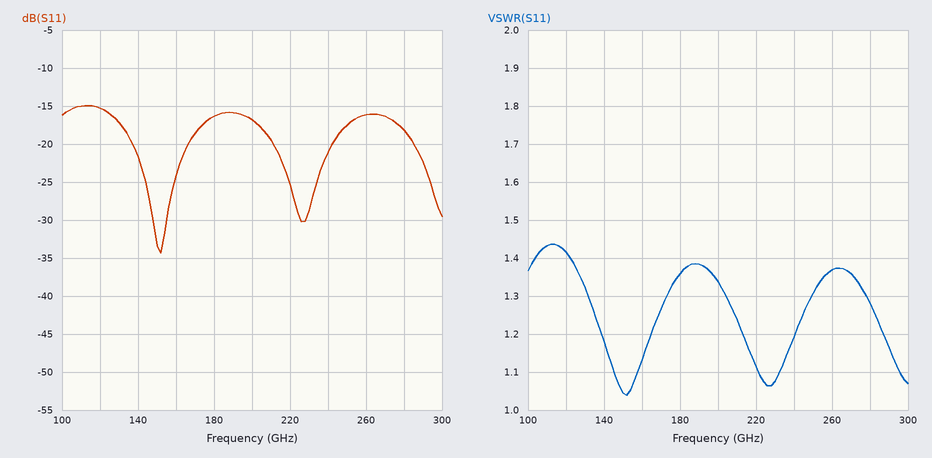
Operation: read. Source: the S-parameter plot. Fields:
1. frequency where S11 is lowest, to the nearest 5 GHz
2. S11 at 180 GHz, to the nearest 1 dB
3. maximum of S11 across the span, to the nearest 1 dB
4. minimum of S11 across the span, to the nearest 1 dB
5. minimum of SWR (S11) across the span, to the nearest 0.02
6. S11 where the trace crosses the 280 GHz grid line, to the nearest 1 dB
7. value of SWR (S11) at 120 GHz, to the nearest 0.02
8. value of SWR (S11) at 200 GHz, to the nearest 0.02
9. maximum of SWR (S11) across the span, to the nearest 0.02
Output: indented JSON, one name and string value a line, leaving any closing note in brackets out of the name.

{
  "frequency where S11 is lowest, to the nearest 5 GHz": "150 GHz",
  "S11 at 180 GHz, to the nearest 1 dB": "-16 dB",
  "maximum of S11 across the span, to the nearest 1 dB": "-15 dB",
  "minimum of S11 across the span, to the nearest 1 dB": "-34 dB",
  "minimum of SWR (S11) across the span, to the nearest 0.02": "1.04",
  "S11 where the trace crosses the 280 GHz grid line, to the nearest 1 dB": "-18 dB",
  "value of SWR (S11) at 120 GHz, to the nearest 0.02": "1.42",
  "value of SWR (S11) at 200 GHz, to the nearest 0.02": "1.34",
  "maximum of SWR (S11) across the span, to the nearest 0.02": "1.44"
}
